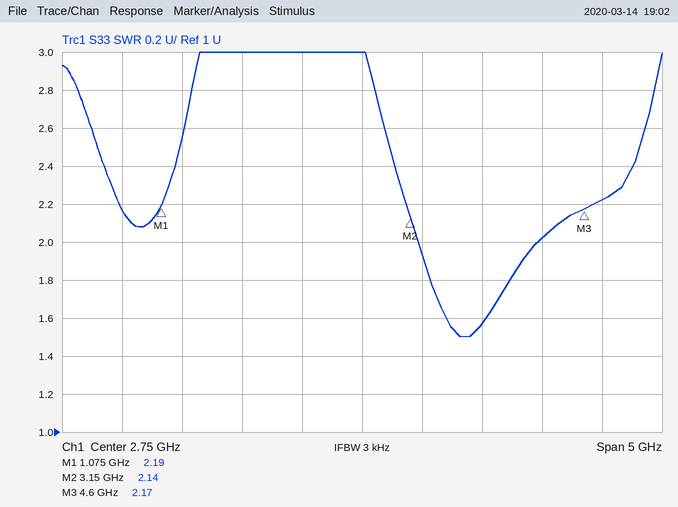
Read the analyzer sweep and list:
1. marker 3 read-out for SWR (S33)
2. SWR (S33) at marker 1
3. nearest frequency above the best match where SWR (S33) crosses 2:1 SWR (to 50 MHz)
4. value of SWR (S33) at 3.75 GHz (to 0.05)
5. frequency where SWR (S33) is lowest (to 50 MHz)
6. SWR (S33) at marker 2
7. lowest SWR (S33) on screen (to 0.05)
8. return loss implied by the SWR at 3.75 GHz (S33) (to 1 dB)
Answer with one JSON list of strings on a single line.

["2.17", "2.19", "4.20 GHz", "1.55", "3.55 GHz", "2.14", "1.50", "13 dB"]
